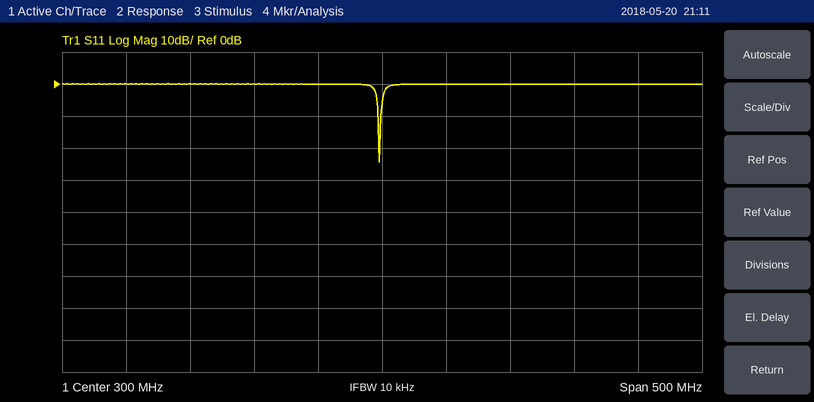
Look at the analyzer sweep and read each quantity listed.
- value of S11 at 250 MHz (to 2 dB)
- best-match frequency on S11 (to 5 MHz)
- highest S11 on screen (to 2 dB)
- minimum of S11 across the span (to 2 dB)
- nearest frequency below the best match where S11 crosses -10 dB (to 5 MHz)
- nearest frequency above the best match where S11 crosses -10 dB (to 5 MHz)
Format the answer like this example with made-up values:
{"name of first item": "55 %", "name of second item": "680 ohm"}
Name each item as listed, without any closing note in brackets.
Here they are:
{"value of S11 at 250 MHz": "0 dB", "best-match frequency on S11": "300 MHz", "highest S11 on screen": "0 dB", "minimum of S11 across the span": "-24 dB", "nearest frequency below the best match where S11 crosses -10 dB": "295 MHz", "nearest frequency above the best match where S11 crosses -10 dB": "300 MHz"}
